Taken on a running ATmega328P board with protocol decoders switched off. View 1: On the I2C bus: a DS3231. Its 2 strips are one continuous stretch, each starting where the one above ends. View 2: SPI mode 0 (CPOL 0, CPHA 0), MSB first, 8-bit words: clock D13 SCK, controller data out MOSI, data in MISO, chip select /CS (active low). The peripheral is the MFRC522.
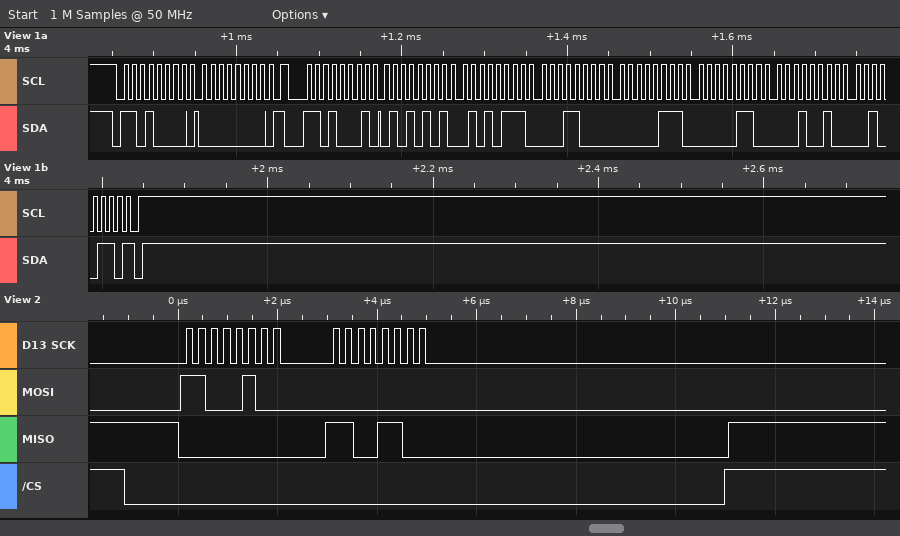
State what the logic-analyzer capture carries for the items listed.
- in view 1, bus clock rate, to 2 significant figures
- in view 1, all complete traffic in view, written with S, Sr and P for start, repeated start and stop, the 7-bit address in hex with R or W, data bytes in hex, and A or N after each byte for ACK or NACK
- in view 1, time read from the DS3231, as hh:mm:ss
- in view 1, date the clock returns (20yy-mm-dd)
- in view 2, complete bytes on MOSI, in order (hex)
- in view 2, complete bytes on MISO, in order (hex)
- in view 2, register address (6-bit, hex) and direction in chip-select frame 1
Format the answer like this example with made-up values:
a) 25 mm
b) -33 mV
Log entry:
a) 100 kHz
b) S 68W A 00 A Sr 68R A 55 A 57 A 18 A 07 A 06 A 12 A 26 N P
c) 18:57:55
d) 2026-12-06
e) 0xC4 0x00
f) 0x00 0xCC
g) 0x22 read
